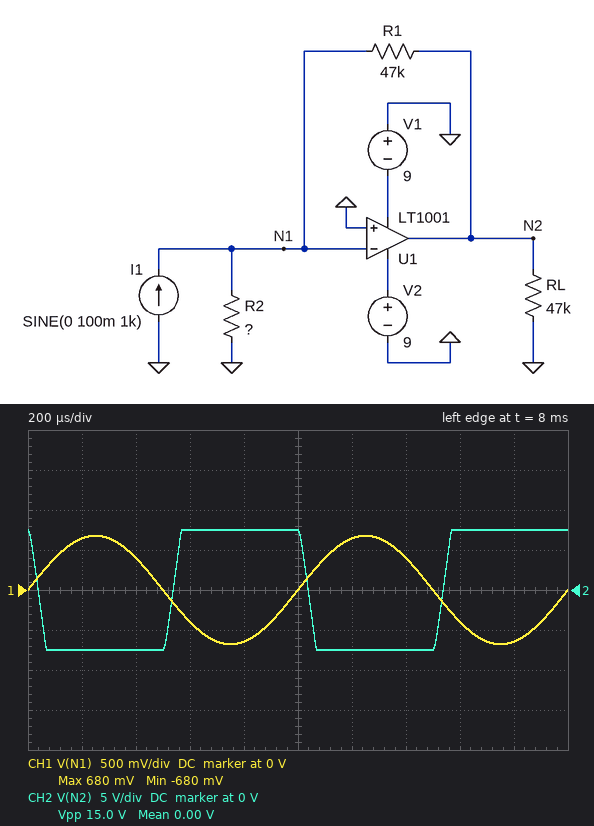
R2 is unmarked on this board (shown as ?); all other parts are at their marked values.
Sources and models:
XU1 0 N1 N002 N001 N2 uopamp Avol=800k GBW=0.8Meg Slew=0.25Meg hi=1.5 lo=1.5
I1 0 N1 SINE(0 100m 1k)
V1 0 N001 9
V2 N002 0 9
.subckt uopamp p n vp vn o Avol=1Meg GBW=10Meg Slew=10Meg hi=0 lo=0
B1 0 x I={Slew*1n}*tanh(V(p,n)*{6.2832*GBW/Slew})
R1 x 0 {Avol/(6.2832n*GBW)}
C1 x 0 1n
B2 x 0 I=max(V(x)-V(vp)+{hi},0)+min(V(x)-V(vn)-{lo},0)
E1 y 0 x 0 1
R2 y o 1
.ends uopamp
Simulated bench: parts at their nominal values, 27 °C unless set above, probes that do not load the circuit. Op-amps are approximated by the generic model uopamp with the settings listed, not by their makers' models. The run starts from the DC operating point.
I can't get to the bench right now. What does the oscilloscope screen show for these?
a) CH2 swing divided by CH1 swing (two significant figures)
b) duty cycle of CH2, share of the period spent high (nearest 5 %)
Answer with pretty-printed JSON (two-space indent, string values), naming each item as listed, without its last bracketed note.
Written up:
{
  "CH2 swing divided by CH1 swing": "11",
  "duty cycle of CH2, share of the period spent high": "50 %"
}
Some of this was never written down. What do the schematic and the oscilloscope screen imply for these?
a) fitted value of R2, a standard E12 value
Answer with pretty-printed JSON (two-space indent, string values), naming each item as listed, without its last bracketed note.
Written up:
{
  "fitted value of R2, a standard E12 value": "6.8 Ω"
}
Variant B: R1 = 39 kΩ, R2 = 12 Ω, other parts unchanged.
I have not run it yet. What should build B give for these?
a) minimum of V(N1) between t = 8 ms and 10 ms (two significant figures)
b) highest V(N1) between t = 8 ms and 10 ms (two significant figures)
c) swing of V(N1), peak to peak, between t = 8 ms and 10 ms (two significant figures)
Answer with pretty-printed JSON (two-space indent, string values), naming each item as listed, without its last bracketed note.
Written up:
{
  "minimum of V(N1) between t = 8 ms and 10 ms": "-1.2 V",
  "highest V(N1) between t = 8 ms and 10 ms": "1.2 V",
  "swing of V(N1), peak to peak, between t = 8 ms and 10 ms": "2.4 V"
}
